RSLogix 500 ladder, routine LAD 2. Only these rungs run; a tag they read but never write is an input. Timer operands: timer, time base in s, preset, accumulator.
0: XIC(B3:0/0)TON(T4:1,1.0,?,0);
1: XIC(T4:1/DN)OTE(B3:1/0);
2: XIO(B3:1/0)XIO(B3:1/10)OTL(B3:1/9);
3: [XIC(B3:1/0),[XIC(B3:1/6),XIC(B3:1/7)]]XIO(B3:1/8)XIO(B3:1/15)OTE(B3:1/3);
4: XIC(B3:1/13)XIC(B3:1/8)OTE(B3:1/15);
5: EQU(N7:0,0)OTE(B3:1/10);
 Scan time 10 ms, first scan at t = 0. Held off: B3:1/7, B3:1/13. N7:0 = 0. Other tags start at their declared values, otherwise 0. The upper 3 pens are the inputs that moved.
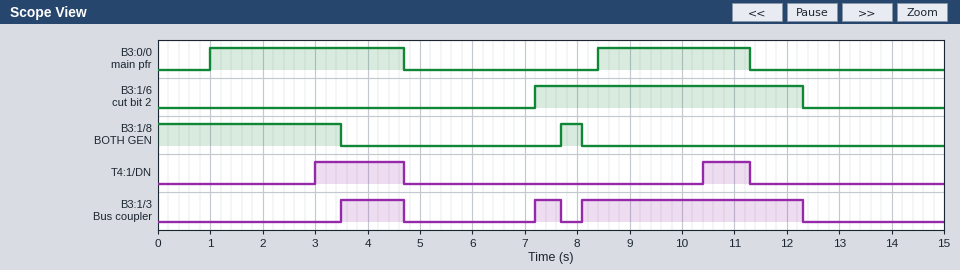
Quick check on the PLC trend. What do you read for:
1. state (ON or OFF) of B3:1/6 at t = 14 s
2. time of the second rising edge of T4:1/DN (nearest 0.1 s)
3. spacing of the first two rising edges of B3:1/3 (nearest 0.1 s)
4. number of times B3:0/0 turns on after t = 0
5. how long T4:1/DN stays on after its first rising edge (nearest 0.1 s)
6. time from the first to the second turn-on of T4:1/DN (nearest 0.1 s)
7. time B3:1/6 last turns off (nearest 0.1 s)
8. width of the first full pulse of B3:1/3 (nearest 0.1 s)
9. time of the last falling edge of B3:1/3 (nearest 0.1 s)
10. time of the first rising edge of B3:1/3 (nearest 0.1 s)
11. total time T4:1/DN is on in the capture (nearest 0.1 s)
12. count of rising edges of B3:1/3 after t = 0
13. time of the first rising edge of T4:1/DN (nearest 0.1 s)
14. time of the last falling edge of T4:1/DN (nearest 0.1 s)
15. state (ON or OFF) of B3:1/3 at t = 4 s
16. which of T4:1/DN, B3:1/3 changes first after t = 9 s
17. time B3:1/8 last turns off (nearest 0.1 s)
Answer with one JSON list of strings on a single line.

["OFF", "10.4 s", "3.7 s", "2", "1.7 s", "7.4 s", "12.3 s", "1.2 s", "12.3 s", "3.5 s", "2.6 s", "3", "3.0 s", "11.3 s", "ON", "T4:1/DN", "8.1 s"]
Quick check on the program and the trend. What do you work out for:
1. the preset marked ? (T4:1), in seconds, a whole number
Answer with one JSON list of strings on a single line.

["2 s"]
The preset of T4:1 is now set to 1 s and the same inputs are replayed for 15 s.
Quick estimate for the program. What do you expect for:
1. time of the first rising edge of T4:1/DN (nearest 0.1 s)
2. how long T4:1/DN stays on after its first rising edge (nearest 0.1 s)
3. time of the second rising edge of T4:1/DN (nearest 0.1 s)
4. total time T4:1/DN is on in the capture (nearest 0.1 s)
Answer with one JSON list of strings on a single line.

["2.0 s", "2.7 s", "9.4 s", "4.6 s"]
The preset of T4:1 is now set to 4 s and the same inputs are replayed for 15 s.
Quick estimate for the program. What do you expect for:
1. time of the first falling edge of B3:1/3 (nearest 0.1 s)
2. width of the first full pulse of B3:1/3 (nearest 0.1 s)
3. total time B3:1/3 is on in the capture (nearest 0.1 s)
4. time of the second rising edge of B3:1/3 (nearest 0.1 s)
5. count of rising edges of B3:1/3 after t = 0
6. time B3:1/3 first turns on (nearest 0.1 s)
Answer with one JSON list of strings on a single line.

["7.7 s", "0.5 s", "4.7 s", "8.1 s", "2", "7.2 s"]
